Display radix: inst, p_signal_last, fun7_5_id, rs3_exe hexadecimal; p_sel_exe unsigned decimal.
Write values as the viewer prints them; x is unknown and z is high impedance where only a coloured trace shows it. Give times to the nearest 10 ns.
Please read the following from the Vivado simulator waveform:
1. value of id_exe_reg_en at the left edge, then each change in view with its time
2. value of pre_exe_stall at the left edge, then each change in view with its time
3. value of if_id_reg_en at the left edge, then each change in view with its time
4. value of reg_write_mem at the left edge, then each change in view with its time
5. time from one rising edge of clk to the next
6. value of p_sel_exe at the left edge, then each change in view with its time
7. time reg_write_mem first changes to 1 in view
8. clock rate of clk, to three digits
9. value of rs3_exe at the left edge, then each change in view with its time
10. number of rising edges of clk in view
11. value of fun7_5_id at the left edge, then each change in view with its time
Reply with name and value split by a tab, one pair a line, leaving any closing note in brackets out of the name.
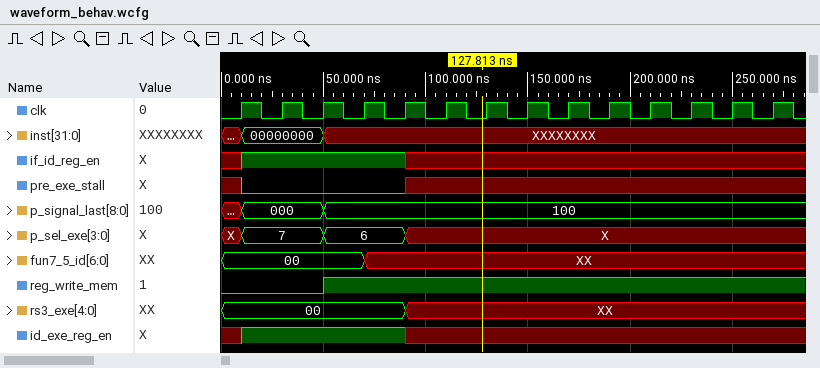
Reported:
value of id_exe_reg_en at the left edge, then each change in view with its time	x, 1 at 10 ns, x at 90 ns
value of pre_exe_stall at the left edge, then each change in view with its time	x, 0 at 10 ns, x at 90 ns
value of if_id_reg_en at the left edge, then each change in view with its time	x, 1 at 10 ns, x at 90 ns
value of reg_write_mem at the left edge, then each change in view with its time	0, 1 at 50 ns
time from one rising edge of clk to the next	20 ns
value of p_sel_exe at the left edge, then each change in view with its time	X, 7 at 10 ns, 6 at 50 ns, X at 90 ns
time reg_write_mem first changes to 1 in view	50 ns
clock rate of clk, to three digits	50.0 MHz
value of rs3_exe at the left edge, then each change in view with its time	00, XX at 90 ns
number of rising edges of clk in view	14
value of fun7_5_id at the left edge, then each change in view with its time	00, XX at 70 ns
